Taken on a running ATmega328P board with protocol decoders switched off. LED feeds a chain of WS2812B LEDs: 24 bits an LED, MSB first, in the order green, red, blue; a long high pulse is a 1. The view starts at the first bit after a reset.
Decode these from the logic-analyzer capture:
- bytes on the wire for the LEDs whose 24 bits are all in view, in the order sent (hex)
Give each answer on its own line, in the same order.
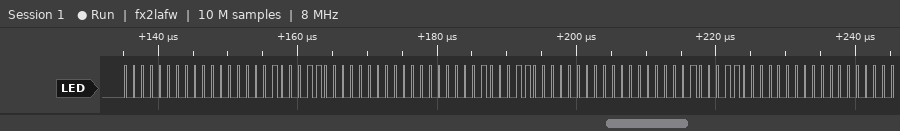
00 00 46 00 00 46 00 00 46
